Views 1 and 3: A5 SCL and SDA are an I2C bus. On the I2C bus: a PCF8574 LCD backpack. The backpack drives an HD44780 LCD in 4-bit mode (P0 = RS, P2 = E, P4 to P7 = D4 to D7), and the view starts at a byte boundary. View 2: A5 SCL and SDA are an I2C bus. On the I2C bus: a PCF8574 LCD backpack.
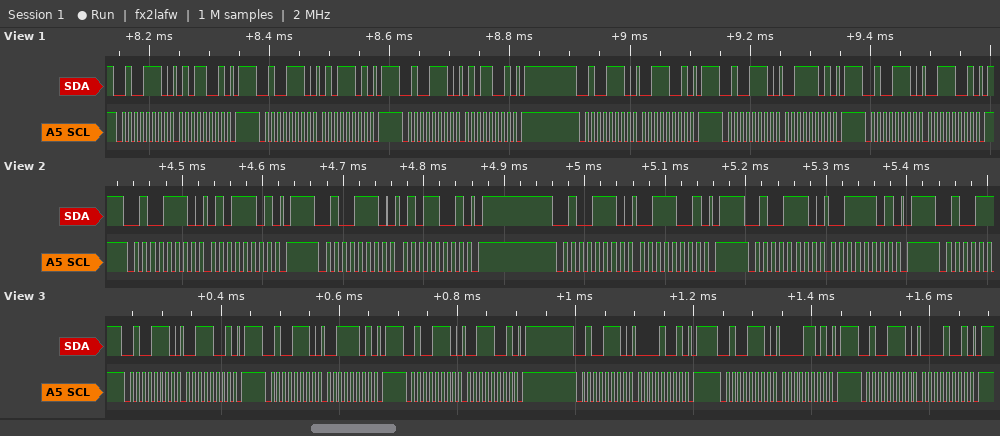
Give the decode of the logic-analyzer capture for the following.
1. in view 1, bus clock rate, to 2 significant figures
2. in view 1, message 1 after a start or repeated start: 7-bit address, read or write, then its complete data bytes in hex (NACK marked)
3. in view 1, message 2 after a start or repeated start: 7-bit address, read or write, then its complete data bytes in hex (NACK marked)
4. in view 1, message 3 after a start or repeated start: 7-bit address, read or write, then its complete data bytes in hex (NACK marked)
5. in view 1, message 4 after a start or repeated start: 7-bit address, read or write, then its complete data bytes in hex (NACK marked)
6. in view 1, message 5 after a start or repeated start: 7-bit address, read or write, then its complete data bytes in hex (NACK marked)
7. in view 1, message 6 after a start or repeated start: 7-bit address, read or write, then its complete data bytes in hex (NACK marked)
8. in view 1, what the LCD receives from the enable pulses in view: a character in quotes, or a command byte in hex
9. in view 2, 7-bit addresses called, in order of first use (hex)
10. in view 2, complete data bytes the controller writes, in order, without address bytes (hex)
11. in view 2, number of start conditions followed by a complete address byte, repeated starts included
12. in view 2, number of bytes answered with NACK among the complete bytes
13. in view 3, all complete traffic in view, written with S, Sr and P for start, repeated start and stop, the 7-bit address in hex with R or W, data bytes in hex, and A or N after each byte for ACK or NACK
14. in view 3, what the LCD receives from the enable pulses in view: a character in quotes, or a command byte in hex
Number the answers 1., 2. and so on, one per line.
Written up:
1. 100 kHz
2. 0x27 write: 59
3. 0x27 write: 5D
4. 0x27 write: 59
5. 0x27 write: 39
6. 0x27 write: 3D
7. 0x27 write: 39
8. 'S'
9. 0x27
10. 5D 59 39 3D
11. 4
12. 0
13. S 27W A 39 A P S 27W A 3D A P S 27W A 39 A P S 27W A 09 A P S 27W A 0D A P S 27W A 09 A P
14. '0'
